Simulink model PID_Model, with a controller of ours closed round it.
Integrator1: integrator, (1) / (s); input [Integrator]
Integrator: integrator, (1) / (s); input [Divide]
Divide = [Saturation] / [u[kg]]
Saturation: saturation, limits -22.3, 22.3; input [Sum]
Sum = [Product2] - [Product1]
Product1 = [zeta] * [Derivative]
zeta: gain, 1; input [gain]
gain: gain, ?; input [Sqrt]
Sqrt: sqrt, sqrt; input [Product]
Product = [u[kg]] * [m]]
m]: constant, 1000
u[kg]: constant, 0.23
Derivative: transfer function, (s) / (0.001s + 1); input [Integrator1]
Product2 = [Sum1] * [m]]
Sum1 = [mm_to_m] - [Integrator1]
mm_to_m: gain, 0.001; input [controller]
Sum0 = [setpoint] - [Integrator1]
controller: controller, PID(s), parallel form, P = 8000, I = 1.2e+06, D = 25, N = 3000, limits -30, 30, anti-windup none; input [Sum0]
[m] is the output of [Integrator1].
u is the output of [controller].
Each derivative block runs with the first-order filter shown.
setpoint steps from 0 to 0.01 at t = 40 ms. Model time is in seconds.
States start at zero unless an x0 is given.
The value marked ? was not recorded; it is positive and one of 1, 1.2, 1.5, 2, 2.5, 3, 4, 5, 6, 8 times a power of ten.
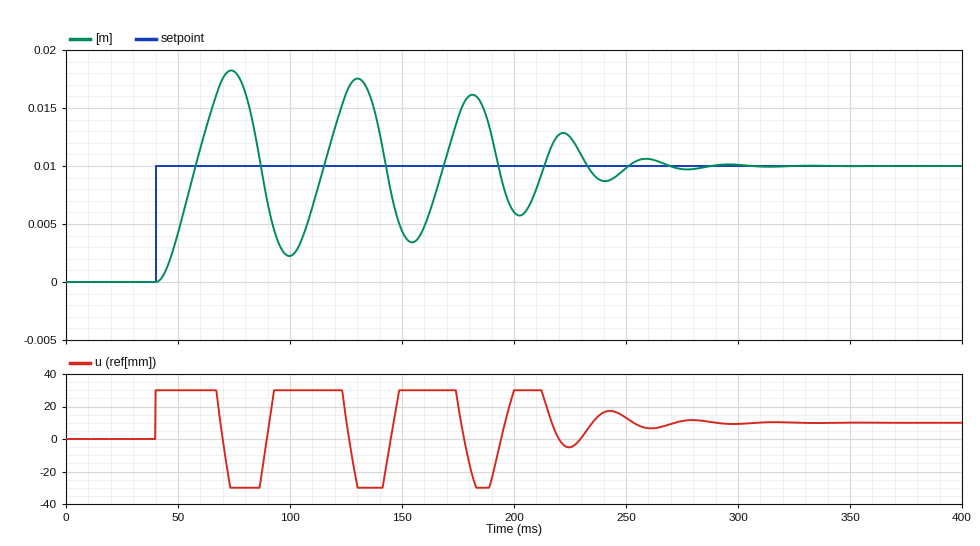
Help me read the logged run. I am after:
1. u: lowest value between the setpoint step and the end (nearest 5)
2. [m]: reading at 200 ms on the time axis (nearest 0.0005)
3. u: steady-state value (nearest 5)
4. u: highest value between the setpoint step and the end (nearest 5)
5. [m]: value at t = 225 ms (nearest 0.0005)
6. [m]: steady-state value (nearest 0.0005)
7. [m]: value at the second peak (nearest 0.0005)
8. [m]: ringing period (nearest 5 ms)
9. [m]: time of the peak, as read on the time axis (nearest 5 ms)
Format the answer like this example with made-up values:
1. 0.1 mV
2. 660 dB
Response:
1. -30
2. 0.0060
3. 10
4. 30
5. 0.0125
6. 0.0100
7. 0.0175
8. 55 ms
9. 75 ms
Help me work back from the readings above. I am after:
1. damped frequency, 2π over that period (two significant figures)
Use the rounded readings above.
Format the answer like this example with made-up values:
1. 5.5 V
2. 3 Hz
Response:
1. 0.11 rad/ms
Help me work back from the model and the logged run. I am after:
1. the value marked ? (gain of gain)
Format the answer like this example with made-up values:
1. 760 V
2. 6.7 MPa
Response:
1. 2
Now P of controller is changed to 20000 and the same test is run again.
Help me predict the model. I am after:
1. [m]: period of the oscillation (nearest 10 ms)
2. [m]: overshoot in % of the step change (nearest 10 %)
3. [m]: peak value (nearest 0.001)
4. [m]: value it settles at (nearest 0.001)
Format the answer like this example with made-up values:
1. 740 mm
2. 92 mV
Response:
1. 30 ms
2. 60 %
3. 0.016
4. 0.010
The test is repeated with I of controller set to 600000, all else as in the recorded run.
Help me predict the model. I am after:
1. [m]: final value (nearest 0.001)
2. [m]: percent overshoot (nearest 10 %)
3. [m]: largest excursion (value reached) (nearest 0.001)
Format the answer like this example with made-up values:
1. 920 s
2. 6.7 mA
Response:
1. 0.010
2. 50 %
3. 0.015
